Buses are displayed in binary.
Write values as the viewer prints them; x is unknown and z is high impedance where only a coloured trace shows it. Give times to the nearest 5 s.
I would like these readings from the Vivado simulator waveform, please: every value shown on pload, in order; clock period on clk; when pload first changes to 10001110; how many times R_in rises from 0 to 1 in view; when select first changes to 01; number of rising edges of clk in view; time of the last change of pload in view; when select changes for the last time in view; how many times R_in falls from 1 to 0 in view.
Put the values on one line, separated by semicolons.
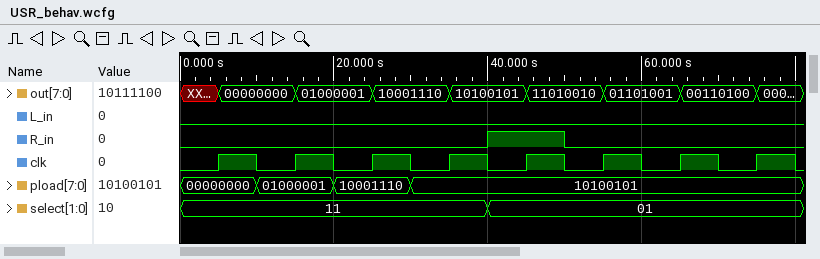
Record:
00000000, 01000001, 10001110, 10100101; 10 s; 20 s; 1; 40 s; 8; 30 s; 40 s; 1
